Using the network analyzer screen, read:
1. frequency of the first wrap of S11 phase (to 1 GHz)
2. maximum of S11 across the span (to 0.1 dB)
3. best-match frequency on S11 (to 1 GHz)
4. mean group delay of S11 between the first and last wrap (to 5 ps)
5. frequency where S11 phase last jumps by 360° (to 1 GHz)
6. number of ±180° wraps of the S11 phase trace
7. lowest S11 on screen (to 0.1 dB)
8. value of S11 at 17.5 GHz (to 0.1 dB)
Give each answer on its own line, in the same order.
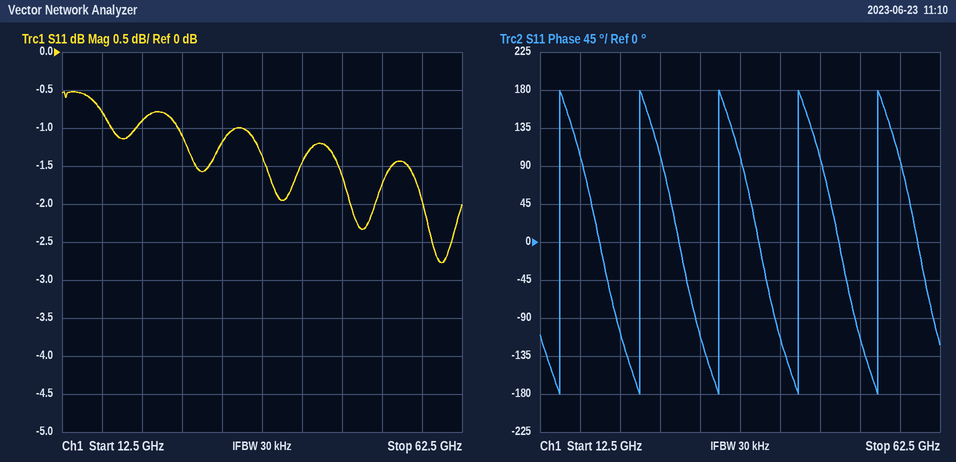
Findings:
15 GHz
-0.5 dB
60 GHz
100 ps
55 GHz
5
-2.8 dB
-0.8 dB
